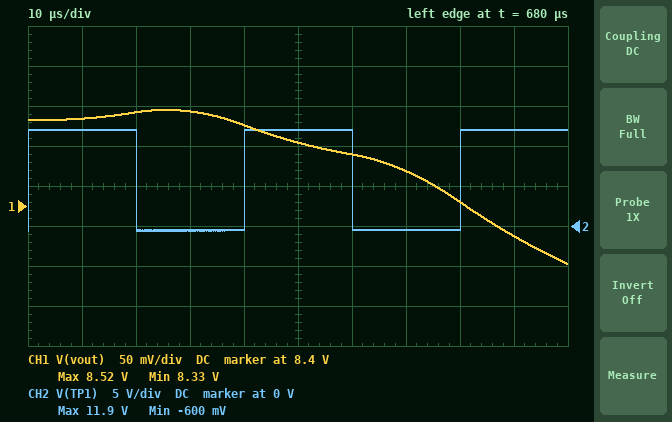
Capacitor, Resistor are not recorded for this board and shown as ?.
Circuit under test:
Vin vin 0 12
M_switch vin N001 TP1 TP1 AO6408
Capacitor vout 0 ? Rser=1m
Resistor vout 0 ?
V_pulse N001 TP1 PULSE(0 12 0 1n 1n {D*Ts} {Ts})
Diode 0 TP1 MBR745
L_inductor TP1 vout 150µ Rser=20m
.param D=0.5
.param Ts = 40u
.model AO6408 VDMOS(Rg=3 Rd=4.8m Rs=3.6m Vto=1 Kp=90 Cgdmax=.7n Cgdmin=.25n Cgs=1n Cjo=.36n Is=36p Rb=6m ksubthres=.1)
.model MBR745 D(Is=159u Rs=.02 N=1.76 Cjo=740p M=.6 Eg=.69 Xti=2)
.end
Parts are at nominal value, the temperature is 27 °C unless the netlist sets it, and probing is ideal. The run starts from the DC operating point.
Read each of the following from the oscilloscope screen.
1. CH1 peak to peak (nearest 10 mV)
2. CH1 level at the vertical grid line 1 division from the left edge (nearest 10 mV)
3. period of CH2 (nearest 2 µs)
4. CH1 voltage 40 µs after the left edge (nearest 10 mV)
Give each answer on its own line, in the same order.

190 mV
8.51 V
40 µs
8.50 V
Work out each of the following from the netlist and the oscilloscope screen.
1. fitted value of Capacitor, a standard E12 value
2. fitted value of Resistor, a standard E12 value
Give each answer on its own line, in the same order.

330 µF
1.8 Ω
